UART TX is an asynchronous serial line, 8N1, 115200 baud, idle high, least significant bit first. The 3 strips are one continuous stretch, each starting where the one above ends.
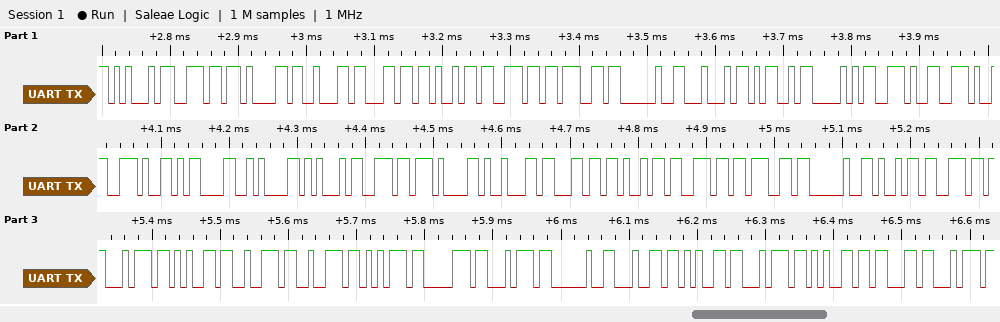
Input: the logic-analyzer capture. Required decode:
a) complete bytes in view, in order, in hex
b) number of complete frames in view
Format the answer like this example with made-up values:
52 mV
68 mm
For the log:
45 6E 61 62 6C 69 6E 67 20 44 4D 50 2E 2E 2E 0D 0A 45 6E 61 62 6C 69 6E 67 20 69 6E 74 65 72 72 75 70 74 20 64 65 74 65 63 74
42
